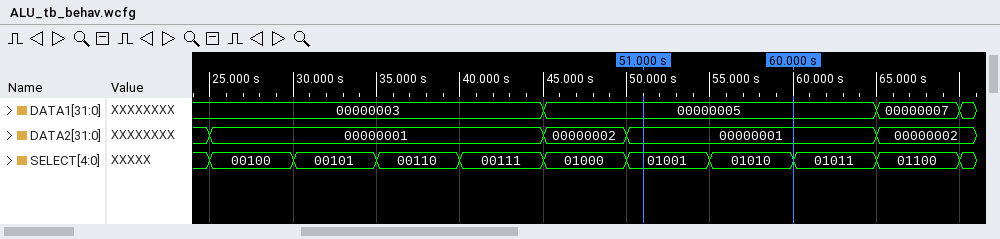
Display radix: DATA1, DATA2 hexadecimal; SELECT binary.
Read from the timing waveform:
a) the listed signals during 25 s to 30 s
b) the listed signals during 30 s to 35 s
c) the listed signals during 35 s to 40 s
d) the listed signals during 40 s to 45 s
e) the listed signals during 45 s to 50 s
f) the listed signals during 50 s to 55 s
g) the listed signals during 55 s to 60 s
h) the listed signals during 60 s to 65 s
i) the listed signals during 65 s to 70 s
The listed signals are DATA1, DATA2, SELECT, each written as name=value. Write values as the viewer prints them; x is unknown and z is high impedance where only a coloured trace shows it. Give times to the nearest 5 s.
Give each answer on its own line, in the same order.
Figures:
DATA1=00000003, DATA2=00000001, SELECT=00100
DATA1=00000003, DATA2=00000001, SELECT=00101
DATA1=00000003, DATA2=00000001, SELECT=00110
DATA1=00000003, DATA2=00000001, SELECT=00111
DATA1=00000005, DATA2=00000002, SELECT=01000
DATA1=00000005, DATA2=00000001, SELECT=01001
DATA1=00000005, DATA2=00000001, SELECT=01010
DATA1=00000005, DATA2=00000001, SELECT=01011
DATA1=00000007, DATA2=00000002, SELECT=01100
